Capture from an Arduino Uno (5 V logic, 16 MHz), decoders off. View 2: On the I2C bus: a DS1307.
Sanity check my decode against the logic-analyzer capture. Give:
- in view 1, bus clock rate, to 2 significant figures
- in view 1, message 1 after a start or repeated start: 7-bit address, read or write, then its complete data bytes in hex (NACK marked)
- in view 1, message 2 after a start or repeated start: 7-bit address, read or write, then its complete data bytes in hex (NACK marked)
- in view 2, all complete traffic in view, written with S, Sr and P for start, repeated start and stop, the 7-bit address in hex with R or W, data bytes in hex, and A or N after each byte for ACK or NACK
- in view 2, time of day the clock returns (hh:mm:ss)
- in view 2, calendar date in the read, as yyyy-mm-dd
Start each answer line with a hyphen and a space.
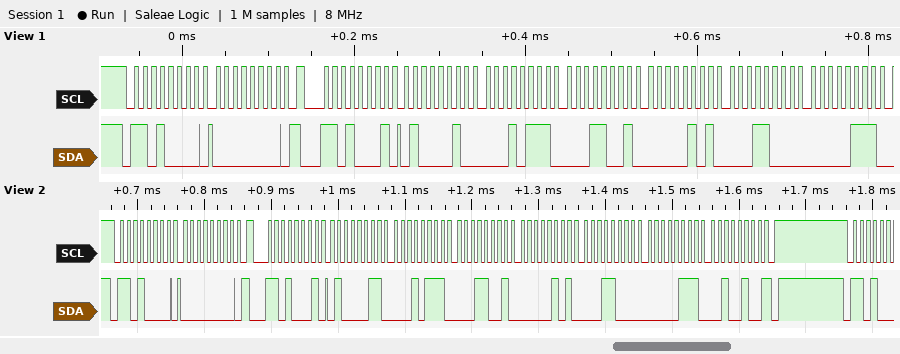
- 100 kHz
- 0x68 write: 00
- 0x68 read: 42 17 19 05 18 07
- S 68W A 00 A Sr 68R A 43 A 17 A 19 A 05 A 18 A 07 A 24 N P
- 19:17:43
- 2024-07-18
